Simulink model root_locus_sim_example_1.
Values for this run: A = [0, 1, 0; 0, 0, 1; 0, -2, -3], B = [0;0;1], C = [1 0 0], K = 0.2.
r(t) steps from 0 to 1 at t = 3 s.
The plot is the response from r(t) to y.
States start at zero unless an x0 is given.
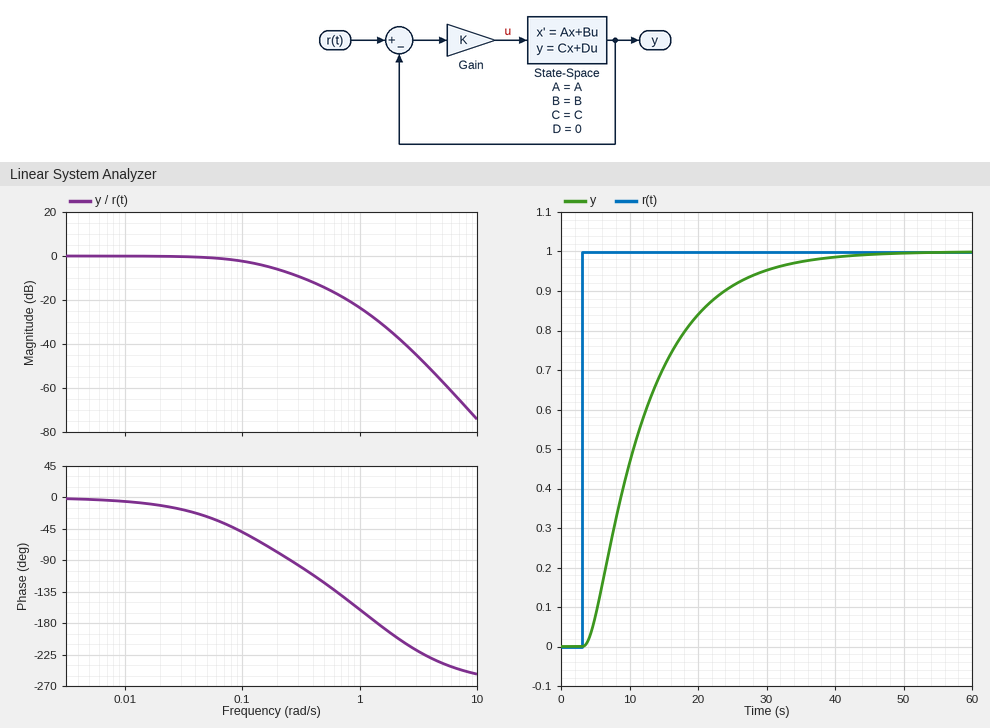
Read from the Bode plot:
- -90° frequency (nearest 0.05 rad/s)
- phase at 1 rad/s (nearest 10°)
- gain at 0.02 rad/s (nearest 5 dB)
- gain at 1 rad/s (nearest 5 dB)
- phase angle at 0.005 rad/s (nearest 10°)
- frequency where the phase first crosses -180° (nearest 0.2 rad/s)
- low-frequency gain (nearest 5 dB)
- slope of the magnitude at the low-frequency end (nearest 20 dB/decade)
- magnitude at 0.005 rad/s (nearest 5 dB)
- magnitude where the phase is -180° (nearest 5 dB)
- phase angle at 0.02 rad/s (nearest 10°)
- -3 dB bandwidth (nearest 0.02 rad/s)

0.25 rad/s
-160°
0 dB
-25 dB
0°
1.4 rad/s
0 dB
0 dB/decade
0 dB
-30 dB
-10°
0.12 rad/s
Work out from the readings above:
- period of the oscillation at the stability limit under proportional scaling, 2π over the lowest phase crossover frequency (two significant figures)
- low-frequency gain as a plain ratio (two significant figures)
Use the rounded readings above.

4.5 s
1.0
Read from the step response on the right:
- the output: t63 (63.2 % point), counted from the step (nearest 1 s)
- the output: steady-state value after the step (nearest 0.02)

10 s
1.00
